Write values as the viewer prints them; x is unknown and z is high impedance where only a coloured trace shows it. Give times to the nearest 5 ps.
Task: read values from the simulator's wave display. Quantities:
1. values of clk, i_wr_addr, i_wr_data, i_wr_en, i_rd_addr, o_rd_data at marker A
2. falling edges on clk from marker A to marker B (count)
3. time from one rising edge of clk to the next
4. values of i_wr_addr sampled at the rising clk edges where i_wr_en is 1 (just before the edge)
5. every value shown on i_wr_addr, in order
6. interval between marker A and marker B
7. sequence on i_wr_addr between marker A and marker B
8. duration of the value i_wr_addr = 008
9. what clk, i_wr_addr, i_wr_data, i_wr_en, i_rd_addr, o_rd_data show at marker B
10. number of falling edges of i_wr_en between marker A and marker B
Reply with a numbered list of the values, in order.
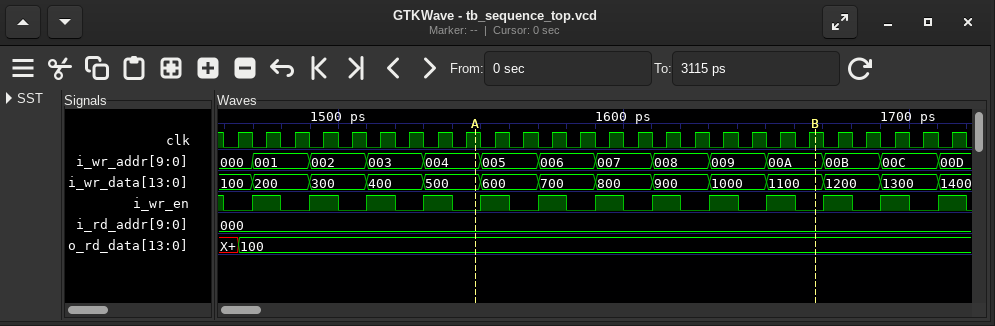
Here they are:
1. clk=1, i_wr_addr=004, i_wr_data=500, i_wr_en=0, i_rd_addr=000, o_rd_data=100
2. 12
3. 10 ps
4. 001, 002, 003, 004, 005, 006, 007, 008, 009, 00A, 00B, 00C, 00D
5. 000, 001, 002, 003, 004, 005, 006, 007, 008, 009, 00A, 00B, 00C, 00D
6. 120 ps
7. 004, 005, 006, 007, 008, 009, 00A
8. 20 ps
9. clk=1, i_wr_addr=00A, i_wr_data=1100, i_wr_en=0, i_rd_addr=000, o_rd_data=100
10. 6
